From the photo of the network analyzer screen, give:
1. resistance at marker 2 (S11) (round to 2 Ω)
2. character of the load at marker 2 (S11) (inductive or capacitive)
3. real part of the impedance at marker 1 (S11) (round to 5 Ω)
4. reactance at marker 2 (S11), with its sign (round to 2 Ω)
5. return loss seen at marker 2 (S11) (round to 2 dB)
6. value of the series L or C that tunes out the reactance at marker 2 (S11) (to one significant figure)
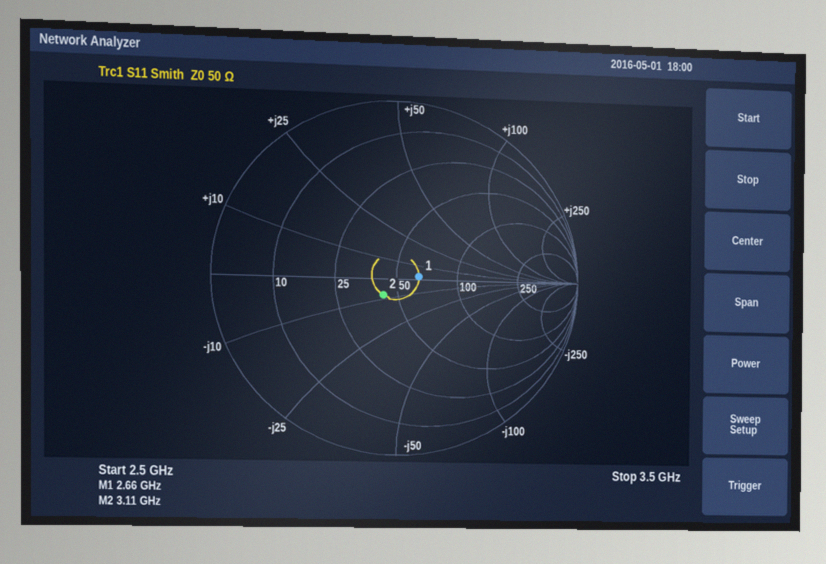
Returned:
42 Ω
capacitive
65 Ω
-8 Ω
18 dB
400 pH
